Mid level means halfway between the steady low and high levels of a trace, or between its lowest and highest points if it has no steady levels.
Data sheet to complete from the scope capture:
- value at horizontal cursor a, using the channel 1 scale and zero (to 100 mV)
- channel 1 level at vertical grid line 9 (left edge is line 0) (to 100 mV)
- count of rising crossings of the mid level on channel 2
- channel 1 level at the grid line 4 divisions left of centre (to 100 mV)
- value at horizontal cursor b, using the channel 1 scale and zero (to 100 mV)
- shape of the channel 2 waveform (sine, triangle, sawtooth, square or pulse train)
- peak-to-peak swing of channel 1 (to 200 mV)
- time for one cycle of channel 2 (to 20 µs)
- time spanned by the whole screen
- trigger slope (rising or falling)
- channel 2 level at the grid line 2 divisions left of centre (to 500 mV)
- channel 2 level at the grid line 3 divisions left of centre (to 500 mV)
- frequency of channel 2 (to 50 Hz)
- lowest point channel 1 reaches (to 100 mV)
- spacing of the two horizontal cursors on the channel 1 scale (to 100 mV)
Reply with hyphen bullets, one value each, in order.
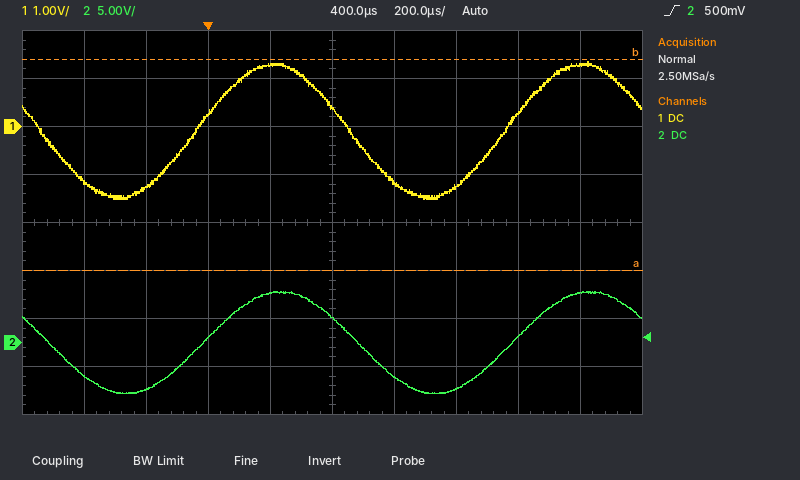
- -3.0 V
- 1.3 V
- 2
- -1.1 V
- 1.4 V
- sine
- 2.8 V
- 1.00 ms
- 2 ms
- rising
- 500 mV
- -5.0 V
- 1.00 kHz
- -1.5 V
- 4.4 V
